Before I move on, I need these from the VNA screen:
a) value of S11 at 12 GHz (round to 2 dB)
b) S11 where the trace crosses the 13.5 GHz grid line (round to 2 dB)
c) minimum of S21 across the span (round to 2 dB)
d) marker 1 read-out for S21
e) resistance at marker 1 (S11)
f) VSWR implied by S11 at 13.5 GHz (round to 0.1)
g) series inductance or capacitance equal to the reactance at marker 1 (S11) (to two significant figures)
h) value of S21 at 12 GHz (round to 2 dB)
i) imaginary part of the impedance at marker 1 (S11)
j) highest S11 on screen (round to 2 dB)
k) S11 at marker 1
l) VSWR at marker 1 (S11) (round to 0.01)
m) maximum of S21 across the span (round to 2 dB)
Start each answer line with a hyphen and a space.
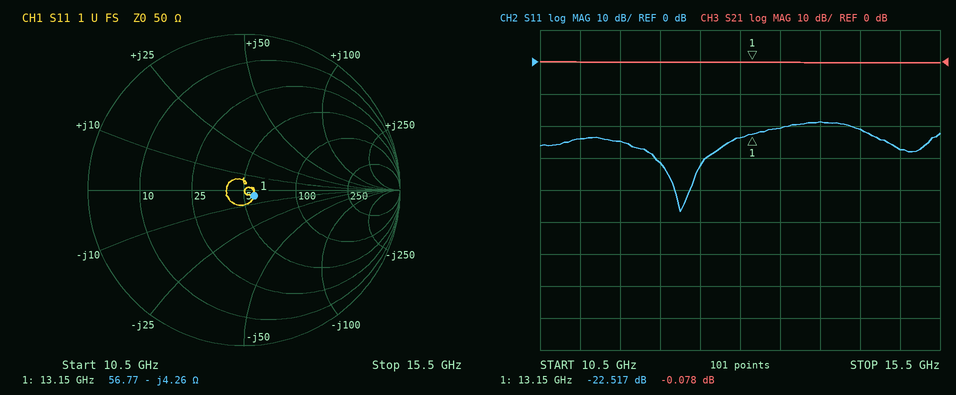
- -32 dB
- -20 dB
- 0 dB
- -0.078 dB
- 56.77 Ω
- 1.2
- 2.8 pF
- 0 dB
- -4.26 Ω
- -18 dB
- -22.517 dB
- 1.16
- 0 dB
